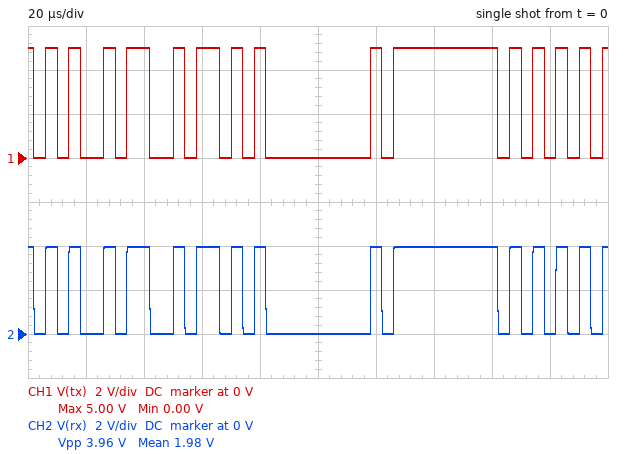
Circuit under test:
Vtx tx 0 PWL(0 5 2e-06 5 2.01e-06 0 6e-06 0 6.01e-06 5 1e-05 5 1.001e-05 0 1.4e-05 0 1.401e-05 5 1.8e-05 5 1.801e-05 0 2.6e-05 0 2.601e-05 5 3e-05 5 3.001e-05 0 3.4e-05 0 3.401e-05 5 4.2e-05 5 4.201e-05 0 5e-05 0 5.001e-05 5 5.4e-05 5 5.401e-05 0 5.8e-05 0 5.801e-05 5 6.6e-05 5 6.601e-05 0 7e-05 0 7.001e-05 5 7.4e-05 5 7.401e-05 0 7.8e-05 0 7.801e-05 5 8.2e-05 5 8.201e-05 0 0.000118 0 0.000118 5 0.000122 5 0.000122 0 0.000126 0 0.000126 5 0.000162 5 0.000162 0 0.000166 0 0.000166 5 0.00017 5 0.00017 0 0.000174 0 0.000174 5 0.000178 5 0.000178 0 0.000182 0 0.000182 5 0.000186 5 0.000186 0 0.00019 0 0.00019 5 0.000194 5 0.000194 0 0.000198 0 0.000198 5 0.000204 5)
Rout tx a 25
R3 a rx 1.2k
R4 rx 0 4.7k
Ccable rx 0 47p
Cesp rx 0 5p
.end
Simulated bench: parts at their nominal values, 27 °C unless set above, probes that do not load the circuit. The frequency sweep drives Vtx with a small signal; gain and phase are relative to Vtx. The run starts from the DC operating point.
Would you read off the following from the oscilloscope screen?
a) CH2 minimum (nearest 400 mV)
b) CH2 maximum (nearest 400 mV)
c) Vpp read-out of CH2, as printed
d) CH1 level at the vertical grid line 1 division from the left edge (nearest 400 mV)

0 V
4.0 V
3.96 V
0 V
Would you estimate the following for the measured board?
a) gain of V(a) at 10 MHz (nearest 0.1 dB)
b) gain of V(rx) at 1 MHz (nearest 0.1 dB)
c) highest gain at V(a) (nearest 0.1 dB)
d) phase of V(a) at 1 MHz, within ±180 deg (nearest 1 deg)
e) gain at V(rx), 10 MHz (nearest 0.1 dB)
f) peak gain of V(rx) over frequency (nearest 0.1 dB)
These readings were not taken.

-0.2 dB
-2.4 dB
0 dB
0 deg
-12.5 dB
-2.0 dB
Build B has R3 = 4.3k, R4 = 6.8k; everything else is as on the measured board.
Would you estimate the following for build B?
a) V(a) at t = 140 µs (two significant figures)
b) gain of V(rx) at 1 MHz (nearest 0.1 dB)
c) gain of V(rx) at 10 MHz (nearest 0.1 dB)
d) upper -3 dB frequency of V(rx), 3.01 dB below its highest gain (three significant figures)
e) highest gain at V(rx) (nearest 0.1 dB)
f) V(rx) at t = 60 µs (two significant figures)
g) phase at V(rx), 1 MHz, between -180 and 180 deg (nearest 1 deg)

5.0 V
-6.7 dB
-23.1 dB
1.16 MHz
-4.3 dB
3.1 V
-41 deg
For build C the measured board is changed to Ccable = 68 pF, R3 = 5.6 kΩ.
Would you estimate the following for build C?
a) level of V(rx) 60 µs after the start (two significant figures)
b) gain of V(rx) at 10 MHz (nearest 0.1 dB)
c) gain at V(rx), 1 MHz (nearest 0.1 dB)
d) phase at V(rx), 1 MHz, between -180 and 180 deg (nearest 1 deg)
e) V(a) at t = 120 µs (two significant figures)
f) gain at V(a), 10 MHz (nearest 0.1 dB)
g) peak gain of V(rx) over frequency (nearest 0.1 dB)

2.3 V
-28.3 dB
-10.6 dB
-50 deg
5.0 V
0 dB
-6.8 dB
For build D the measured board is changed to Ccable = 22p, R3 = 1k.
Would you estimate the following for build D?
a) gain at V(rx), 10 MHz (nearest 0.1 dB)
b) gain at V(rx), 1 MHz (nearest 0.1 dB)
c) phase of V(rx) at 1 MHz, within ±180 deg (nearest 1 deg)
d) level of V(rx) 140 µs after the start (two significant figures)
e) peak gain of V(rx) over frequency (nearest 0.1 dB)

-6.5 dB
-1.8 dB
-8 deg
4.1 V
-1.7 dB
